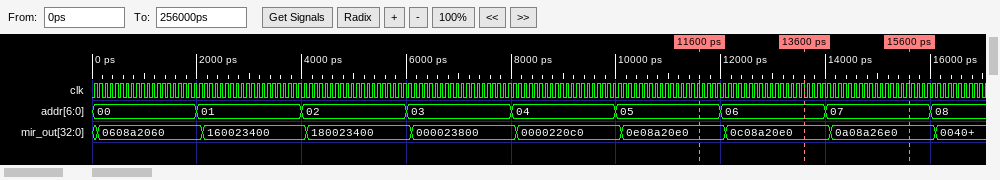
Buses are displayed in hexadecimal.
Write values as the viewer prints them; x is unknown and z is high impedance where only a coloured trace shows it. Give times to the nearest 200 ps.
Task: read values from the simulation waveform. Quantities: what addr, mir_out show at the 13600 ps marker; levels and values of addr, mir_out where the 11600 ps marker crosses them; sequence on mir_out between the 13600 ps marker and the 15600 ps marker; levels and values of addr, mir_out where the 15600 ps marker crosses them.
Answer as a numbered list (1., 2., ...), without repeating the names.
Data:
1. addr=06, mir_out=0c08a20e0
2. addr=05, mir_out=0e08a20e0
3. 0c08a20e0, 0a08a26e0
4. addr=07, mir_out=0a08a26e0
